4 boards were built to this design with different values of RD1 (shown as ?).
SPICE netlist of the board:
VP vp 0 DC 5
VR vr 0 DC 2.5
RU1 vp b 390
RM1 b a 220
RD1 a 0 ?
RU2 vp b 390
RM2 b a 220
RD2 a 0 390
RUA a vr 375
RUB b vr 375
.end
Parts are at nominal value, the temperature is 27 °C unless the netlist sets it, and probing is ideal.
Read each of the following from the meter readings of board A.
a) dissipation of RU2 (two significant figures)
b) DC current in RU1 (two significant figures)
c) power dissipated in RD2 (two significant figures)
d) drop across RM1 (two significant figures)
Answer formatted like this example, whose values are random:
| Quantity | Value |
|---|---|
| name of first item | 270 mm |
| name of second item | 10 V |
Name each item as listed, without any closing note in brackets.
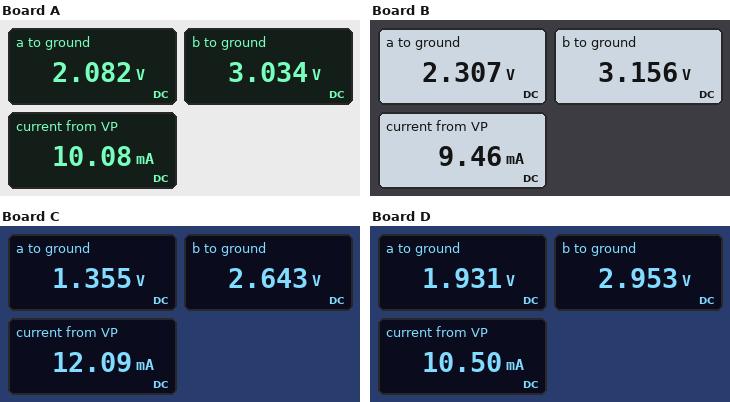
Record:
| Quantity | Value |
|---|---|
| dissipation of RU2 | 9.9 mW |
| DC current in RU1 | 5.0 mA |
| power dissipated in RD2 | 11 mW |
| drop across RM1 | 950 mV |
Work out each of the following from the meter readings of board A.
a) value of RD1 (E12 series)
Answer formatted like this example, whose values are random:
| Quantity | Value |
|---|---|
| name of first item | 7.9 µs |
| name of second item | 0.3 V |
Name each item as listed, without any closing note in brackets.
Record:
| Quantity | Value |
|---|---|
| value of RD1 | 470 Ω |
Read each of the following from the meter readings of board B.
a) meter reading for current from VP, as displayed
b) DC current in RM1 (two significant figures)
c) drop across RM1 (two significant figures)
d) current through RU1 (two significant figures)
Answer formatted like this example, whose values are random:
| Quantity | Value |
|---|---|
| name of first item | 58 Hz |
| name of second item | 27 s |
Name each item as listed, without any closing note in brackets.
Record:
| Quantity | Value |
|---|---|
| meter reading for current from VP, as displayed | 9.46 mA |
| DC current in RM1 | 3.9 mA |
| drop across RM1 | 850 mV |
| current through RU1 | 4.7 mA |
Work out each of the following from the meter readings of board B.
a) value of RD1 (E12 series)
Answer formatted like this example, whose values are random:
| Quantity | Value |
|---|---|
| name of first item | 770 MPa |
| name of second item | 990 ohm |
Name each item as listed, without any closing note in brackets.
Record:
| Quantity | Value |
|---|---|
| value of RD1 | 1 kΩ |
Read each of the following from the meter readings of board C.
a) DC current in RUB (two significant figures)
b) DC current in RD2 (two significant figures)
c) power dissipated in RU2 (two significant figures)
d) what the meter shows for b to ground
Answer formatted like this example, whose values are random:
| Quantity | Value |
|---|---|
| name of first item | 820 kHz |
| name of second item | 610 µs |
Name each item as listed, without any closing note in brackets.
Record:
| Quantity | Value |
|---|---|
| DC current in RUB | 380 µA |
| DC current in RD2 | 3.5 mA |
| power dissipated in RU2 | 14 mW |
| what the meter shows for b to ground | 2.643 V |
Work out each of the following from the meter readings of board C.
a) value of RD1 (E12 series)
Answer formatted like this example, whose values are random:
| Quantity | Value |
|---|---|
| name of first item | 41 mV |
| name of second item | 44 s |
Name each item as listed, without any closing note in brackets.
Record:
| Quantity | Value |
|---|---|
| value of RD1 | 120 Ω |
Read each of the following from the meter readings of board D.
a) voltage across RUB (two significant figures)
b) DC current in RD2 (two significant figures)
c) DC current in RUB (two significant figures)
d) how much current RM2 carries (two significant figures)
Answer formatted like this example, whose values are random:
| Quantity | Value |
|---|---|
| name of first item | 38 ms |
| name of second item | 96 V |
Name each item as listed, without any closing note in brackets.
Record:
| Quantity | Value |
|---|---|
| voltage across RUB | 450 mV |
| DC current in RD2 | 5.0 mA |
| DC current in RUB | 1.2 mA |
| how much current RM2 carries | 4.6 mA |
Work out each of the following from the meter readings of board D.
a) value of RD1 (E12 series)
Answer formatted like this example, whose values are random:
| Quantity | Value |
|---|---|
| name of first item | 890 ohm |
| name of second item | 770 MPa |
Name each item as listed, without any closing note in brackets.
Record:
| Quantity | Value |
|---|---|
| value of RD1 | 330 Ω |
